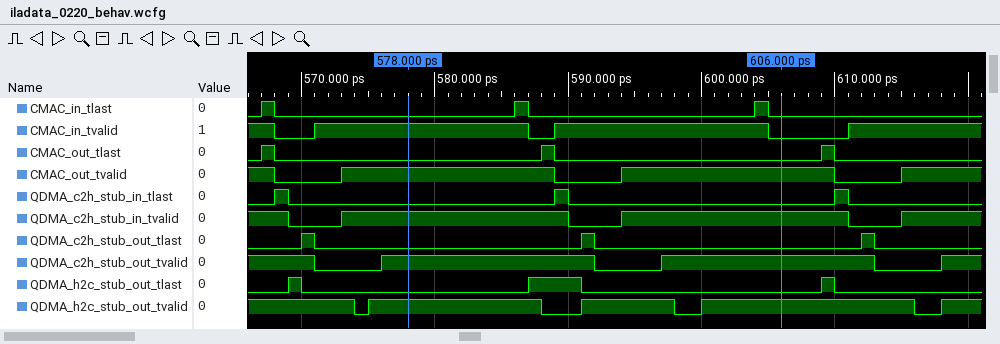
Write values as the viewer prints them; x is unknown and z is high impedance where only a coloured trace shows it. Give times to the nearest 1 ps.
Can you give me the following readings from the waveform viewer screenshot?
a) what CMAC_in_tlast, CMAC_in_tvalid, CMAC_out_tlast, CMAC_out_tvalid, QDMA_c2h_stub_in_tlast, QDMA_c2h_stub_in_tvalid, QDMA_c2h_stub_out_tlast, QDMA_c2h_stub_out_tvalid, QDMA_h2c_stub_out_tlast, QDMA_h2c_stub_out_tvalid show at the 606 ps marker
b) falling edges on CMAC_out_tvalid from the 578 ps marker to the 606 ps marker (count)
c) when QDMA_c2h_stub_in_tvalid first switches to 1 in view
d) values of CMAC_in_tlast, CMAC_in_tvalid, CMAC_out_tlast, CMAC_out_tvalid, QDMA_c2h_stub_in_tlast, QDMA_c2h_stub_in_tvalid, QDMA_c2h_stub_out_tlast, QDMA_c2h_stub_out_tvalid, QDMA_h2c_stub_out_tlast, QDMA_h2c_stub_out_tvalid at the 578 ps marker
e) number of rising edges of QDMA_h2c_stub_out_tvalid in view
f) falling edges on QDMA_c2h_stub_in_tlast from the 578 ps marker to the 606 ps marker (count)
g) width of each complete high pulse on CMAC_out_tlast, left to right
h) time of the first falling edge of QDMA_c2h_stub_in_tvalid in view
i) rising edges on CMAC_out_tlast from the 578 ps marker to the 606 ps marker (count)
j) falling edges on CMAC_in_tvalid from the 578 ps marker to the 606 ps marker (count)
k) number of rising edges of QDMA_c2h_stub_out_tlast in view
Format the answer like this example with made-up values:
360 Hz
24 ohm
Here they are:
CMAC_in_tlast=0, CMAC_in_tvalid=0, CMAC_out_tlast=0, CMAC_out_tvalid=1, QDMA_c2h_stub_in_tlast=0, QDMA_c2h_stub_in_tvalid=1, QDMA_c2h_stub_out_tlast=0, QDMA_c2h_stub_out_tvalid=1, QDMA_h2c_stub_out_tlast=0, QDMA_h2c_stub_out_tvalid=1
1
573 ps
CMAC_in_tlast=0, CMAC_in_tvalid=1, CMAC_out_tlast=0, CMAC_out_tvalid=1, QDMA_c2h_stub_in_tlast=0, QDMA_c2h_stub_in_tvalid=1, QDMA_c2h_stub_out_tlast=0, QDMA_c2h_stub_out_tvalid=1, QDMA_h2c_stub_out_tlast=0, QDMA_h2c_stub_out_tvalid=1
4
1
1 ps, 1 ps, 1 ps
569 ps
1
2
3
